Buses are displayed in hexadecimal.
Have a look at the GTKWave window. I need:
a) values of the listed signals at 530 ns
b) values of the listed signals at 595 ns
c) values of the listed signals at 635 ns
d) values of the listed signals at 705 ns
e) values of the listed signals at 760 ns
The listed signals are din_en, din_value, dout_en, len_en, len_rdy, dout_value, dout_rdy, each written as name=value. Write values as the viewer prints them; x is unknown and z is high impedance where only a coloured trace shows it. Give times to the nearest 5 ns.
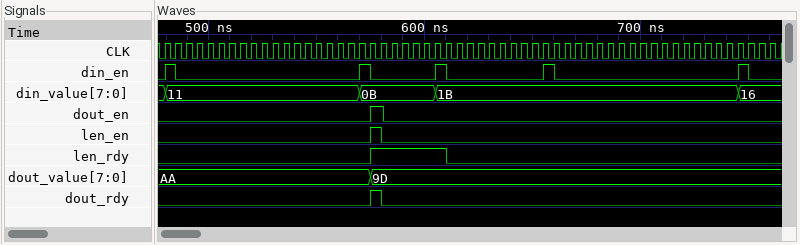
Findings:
din_en=0, din_value=11, dout_en=0, len_en=0, len_rdy=0, dout_value=AA, dout_rdy=0
din_en=0, din_value=0B, dout_en=0, len_en=0, len_rdy=1, dout_value=9D, dout_rdy=0
din_en=0, din_value=1B, dout_en=0, len_en=0, len_rdy=0, dout_value=9D, dout_rdy=0
din_en=0, din_value=1B, dout_en=0, len_en=0, len_rdy=0, dout_value=9D, dout_rdy=0
din_en=0, din_value=16, dout_en=0, len_en=0, len_rdy=0, dout_value=9D, dout_rdy=0
